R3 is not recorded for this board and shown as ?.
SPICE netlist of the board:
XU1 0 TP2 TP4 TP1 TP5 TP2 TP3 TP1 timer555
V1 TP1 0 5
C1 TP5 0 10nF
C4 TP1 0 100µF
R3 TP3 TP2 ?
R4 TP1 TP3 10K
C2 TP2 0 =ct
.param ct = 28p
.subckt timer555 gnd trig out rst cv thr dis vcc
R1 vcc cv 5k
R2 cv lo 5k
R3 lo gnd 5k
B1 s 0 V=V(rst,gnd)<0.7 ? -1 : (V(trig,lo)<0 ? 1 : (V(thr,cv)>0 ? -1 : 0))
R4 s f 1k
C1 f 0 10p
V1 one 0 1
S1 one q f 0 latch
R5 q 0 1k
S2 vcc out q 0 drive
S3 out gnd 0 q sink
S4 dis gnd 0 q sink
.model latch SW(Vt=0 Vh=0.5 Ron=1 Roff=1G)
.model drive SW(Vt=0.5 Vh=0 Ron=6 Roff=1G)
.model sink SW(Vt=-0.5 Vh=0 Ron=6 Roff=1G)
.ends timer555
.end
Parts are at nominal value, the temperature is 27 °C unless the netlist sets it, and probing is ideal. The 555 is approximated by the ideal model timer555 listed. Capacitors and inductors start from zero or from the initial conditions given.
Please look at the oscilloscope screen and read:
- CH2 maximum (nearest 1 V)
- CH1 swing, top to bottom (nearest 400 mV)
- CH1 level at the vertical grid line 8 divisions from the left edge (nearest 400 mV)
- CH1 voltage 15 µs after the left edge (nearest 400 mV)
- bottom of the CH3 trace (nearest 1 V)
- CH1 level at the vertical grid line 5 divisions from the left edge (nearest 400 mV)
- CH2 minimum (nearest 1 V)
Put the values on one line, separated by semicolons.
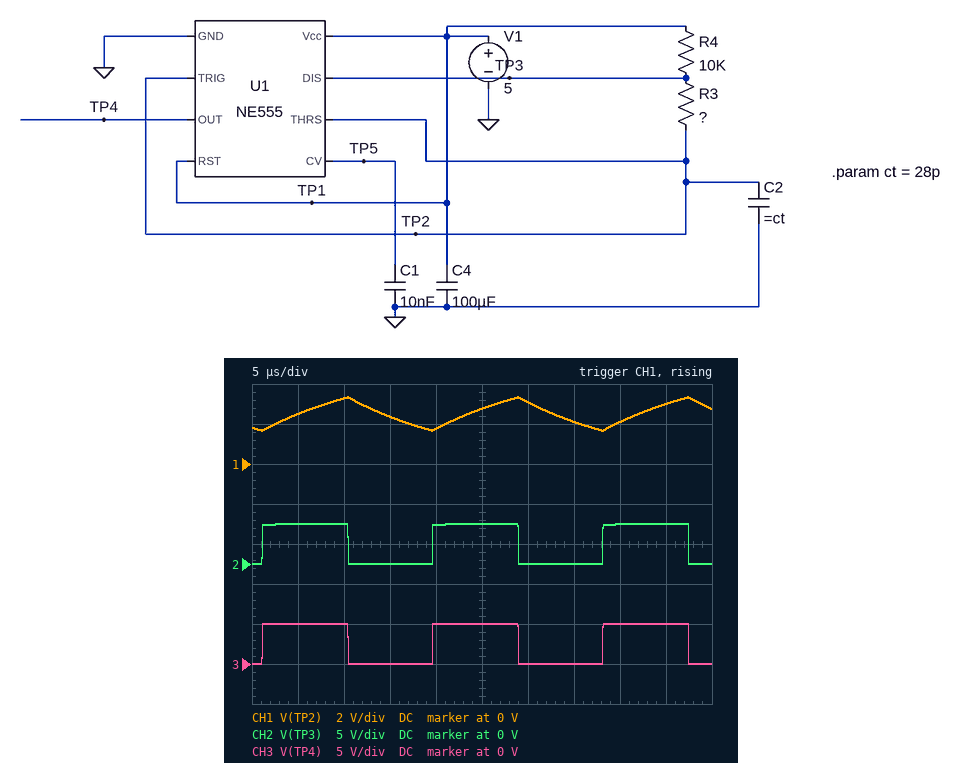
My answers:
5 V; 1.6 V; 2.0 V; 2.4 V; 0 V; 2.8 V; 0 V
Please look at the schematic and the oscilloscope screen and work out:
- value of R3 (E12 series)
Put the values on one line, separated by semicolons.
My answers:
470 kΩ
